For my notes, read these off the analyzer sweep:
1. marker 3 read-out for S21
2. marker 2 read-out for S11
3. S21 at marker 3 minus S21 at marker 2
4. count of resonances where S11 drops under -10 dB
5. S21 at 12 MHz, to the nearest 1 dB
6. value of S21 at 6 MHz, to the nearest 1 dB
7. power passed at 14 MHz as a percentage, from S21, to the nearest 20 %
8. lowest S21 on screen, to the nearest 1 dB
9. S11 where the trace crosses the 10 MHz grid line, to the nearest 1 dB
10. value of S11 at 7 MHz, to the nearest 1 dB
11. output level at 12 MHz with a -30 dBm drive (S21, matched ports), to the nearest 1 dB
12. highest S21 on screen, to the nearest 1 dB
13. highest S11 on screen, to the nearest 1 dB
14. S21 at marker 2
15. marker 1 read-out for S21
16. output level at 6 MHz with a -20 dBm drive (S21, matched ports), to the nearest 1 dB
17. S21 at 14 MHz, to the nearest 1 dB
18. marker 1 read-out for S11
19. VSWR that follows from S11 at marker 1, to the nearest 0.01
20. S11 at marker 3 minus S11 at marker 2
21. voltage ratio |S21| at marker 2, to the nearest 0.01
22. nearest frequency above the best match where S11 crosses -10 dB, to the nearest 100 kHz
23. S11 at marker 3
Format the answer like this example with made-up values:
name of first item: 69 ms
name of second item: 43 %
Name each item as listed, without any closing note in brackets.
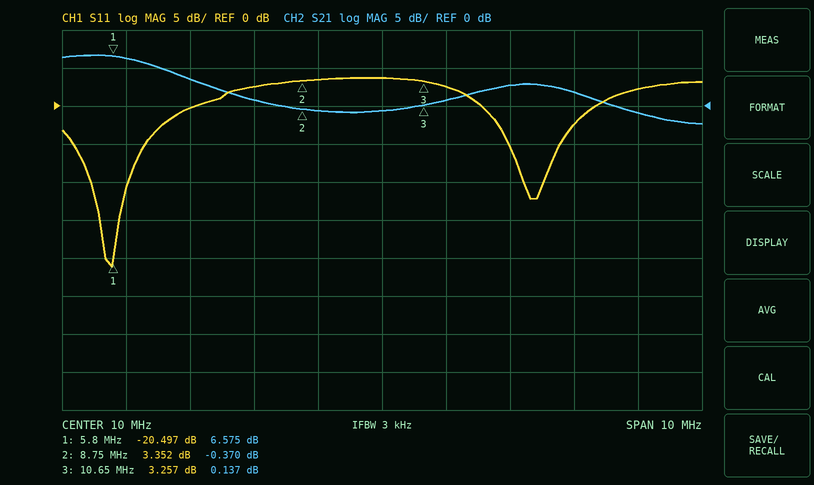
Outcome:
marker 3 read-out for S21: 0.137 dB
marker 2 read-out for S11: 3.352 dB
S21 at marker 3 minus S21 at marker 2: 0.507 dB
count of resonances where S11 drops under -10 dB: 2
S21 at 12 MHz, to the nearest 1 dB: 3 dB
value of S21 at 6 MHz, to the nearest 1 dB: 6 dB
power passed at 14 MHz as a percentage, from S21, to the nearest 20 %: 80 %
lowest S21 on screen, to the nearest 1 dB: -2 dB
S11 where the trace crosses the 10 MHz grid line, to the nearest 1 dB: 4 dB
value of S11 at 7 MHz, to the nearest 1 dB: 0 dB
output level at 12 MHz with a -30 dBm drive (S21, matched ports), to the nearest 1 dB: -27 dBm
highest S21 on screen, to the nearest 1 dB: 7 dB
highest S11 on screen, to the nearest 1 dB: 4 dB
S21 at marker 2: -0.370 dB
marker 1 read-out for S21: 6.575 dB
output level at 6 MHz with a -20 dBm drive (S21, matched ports), to the nearest 1 dB: -14 dBm
S21 at 14 MHz, to the nearest 1 dB: -1 dB
marker 1 read-out for S11: -20.497 dB
VSWR that follows from S11 at marker 1, to the nearest 0.01: 1.21
S11 at marker 3 minus S11 at marker 2: -0.095 dB
voltage ratio |S21| at marker 2, to the nearest 0.01: 0.96
nearest frequency above the best match where S11 crosses -10 dB, to the nearest 100 kHz: 6.0 MHz
S11 at marker 3: 3.257 dB
